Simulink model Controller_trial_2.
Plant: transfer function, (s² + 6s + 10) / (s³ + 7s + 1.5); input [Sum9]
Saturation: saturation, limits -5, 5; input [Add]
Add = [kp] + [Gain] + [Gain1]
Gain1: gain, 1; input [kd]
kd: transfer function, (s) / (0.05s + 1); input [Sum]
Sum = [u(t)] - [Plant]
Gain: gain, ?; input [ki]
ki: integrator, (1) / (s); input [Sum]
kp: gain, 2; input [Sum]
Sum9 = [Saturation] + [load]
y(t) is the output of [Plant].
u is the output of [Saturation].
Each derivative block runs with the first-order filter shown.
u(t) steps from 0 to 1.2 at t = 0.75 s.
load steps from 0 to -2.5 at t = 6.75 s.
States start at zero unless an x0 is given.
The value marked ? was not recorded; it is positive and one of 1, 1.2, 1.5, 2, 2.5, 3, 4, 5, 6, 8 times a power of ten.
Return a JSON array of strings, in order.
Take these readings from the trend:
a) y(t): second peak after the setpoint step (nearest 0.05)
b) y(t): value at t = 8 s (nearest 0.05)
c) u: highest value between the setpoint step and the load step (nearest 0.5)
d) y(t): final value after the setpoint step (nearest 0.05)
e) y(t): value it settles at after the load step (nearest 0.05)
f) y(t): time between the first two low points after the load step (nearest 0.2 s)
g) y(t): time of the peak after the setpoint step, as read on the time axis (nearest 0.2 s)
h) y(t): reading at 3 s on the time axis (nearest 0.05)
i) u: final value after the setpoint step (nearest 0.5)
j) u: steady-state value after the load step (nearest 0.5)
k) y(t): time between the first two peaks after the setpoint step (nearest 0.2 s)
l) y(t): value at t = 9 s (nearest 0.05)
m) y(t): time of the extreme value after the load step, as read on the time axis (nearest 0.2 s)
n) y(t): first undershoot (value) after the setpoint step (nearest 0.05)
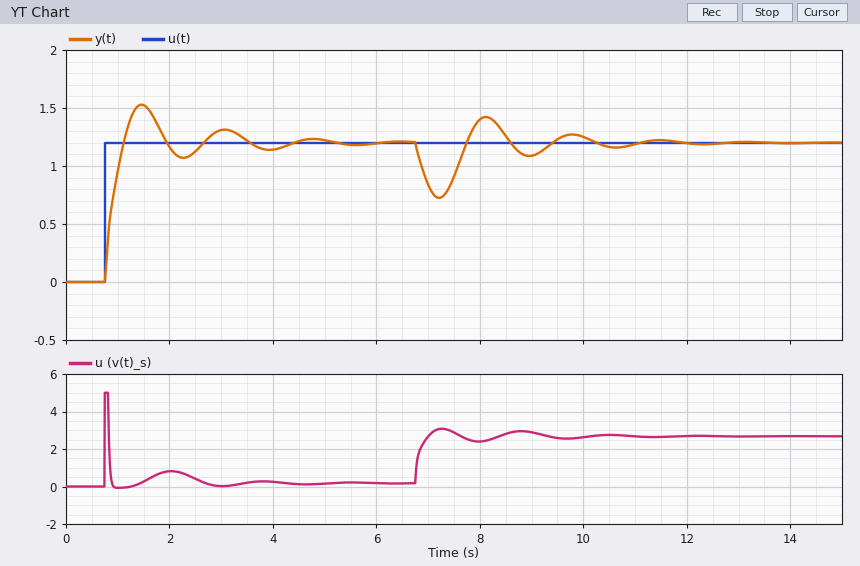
["1.30", "1.40", "5.0", "1.20", "1.20", "1.8 s", "1.4 s", "1.30", "0.0", "2.5", "1.6 s", "1.10", "7.2 s", "1.05"]
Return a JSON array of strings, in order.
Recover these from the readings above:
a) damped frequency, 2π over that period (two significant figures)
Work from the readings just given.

["3.9 rad/s"]
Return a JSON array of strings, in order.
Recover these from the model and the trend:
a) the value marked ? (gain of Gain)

["12"]
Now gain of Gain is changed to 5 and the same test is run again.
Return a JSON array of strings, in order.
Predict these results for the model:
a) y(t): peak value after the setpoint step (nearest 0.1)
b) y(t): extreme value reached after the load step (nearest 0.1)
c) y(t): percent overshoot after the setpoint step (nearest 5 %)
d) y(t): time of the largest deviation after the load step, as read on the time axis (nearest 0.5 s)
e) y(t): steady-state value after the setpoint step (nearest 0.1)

["1.3", "0.6", "10 %", "7.5 s", "1.2"]
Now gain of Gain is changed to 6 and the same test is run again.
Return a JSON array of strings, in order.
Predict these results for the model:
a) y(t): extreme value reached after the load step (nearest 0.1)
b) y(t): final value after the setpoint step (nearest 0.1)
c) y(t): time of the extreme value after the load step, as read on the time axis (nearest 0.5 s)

["0.6", "1.2", "7.5 s"]
